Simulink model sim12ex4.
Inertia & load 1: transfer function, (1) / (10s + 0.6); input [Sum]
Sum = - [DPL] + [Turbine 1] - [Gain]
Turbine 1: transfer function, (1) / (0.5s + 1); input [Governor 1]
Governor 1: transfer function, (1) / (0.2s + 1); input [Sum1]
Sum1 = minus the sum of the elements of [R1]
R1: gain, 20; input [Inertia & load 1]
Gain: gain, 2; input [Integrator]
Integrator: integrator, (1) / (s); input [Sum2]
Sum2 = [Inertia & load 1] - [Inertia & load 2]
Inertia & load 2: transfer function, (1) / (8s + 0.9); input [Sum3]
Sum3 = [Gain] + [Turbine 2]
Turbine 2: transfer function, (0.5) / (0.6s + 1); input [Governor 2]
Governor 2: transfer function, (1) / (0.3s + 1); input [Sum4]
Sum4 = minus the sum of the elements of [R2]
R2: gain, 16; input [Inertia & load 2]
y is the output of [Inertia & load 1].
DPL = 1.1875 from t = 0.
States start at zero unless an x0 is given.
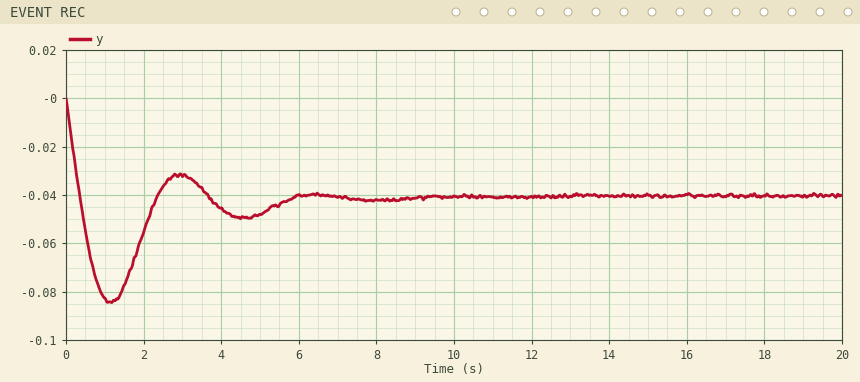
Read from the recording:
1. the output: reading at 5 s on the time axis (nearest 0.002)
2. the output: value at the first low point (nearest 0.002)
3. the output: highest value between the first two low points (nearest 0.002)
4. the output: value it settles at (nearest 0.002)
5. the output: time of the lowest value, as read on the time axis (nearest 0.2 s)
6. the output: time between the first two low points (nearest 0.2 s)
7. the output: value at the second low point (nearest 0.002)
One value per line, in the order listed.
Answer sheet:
-0.048
-0.084
-0.032
-0.040
1.2 s
3.4 s
-0.050
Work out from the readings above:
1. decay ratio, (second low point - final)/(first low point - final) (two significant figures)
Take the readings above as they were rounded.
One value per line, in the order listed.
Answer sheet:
0.23
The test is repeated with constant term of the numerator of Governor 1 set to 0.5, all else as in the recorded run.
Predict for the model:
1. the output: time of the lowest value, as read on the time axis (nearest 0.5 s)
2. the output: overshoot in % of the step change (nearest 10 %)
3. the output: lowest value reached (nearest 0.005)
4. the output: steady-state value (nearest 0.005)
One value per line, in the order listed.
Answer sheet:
1.5 s
90 %
-0.115
-0.060
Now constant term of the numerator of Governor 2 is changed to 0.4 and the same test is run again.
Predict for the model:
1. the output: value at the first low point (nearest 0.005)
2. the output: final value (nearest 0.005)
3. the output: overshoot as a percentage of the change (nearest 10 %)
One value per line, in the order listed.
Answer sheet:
-0.085
-0.050
80 %
